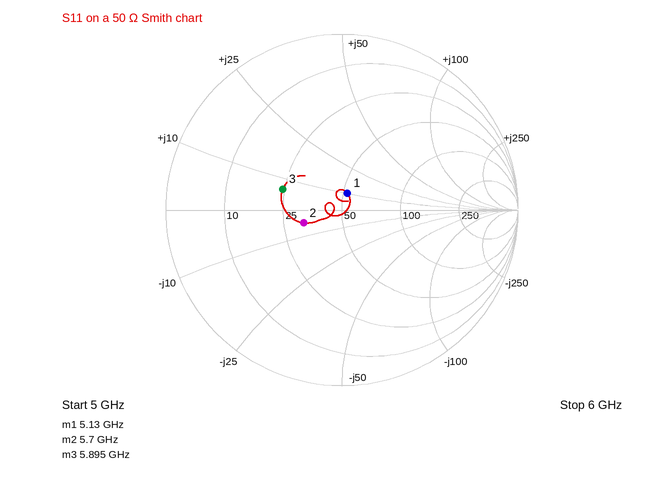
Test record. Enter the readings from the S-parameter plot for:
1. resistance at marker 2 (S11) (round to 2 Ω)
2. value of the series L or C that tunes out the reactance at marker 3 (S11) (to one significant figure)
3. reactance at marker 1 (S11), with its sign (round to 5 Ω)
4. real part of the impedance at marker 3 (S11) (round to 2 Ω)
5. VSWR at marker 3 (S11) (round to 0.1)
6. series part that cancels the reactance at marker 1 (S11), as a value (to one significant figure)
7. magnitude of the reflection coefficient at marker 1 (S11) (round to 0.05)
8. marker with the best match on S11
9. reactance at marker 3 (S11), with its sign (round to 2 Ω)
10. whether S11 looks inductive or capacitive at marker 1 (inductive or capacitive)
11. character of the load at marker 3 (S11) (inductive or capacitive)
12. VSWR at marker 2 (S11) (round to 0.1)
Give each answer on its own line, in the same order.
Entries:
32 Ω
4 pF
+10 Ω
24 Ω
2.1
3 pF
0.10
marker 1
+6 Ω
inductive
inductive
1.6
